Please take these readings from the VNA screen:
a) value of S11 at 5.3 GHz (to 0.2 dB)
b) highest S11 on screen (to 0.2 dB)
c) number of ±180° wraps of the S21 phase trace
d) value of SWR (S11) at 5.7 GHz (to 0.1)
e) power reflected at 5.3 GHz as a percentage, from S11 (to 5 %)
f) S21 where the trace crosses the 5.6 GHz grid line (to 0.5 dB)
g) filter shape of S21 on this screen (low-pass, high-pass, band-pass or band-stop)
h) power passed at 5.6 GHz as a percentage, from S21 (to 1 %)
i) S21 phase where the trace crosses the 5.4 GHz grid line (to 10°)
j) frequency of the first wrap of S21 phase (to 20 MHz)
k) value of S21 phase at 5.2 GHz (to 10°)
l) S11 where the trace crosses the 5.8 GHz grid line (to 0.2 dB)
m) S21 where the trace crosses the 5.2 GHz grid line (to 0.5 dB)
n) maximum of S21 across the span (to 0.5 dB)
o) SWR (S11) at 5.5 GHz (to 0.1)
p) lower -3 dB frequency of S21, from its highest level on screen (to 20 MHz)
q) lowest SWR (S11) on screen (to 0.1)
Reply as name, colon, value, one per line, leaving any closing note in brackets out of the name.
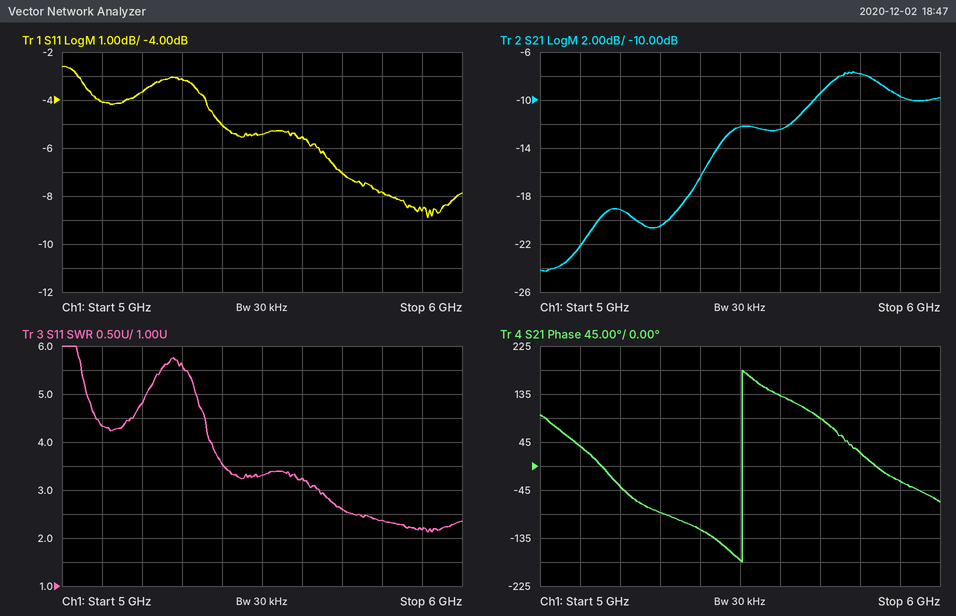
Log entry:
value of S11 at 5.3 GHz: -3.2 dB
highest S11 on screen: -2.6 dB
number of ±180° wraps of the S21 phase trace: 1
value of SWR (S11) at 5.7 GHz: 2.6
power reflected at 5.3 GHz as a percentage, from S11: 50 %
S21 where the trace crosses the 5.6 GHz grid line: -12.5 dB
filter shape of S21 on this screen: high-pass
power passed at 5.6 GHz as a percentage, from S21: 6 %
S21 phase where the trace crosses the 5.4 GHz grid line: -120°
frequency of the first wrap of S21 phase: 5.50 GHz
value of S21 phase at 5.2 GHz: -40°
S11 where the trace crosses the 5.8 GHz grid line: -7.8 dB
S21 where the trace crosses the 5.2 GHz grid line: -19.0 dB
maximum of S21 across the span: -7.5 dB
SWR (S11) at 5.5 GHz: 3.3
lower -3 dB frequency of S21, from its highest level on screen: 5.66 GHz
lowest SWR (S11) on screen: 2.1
